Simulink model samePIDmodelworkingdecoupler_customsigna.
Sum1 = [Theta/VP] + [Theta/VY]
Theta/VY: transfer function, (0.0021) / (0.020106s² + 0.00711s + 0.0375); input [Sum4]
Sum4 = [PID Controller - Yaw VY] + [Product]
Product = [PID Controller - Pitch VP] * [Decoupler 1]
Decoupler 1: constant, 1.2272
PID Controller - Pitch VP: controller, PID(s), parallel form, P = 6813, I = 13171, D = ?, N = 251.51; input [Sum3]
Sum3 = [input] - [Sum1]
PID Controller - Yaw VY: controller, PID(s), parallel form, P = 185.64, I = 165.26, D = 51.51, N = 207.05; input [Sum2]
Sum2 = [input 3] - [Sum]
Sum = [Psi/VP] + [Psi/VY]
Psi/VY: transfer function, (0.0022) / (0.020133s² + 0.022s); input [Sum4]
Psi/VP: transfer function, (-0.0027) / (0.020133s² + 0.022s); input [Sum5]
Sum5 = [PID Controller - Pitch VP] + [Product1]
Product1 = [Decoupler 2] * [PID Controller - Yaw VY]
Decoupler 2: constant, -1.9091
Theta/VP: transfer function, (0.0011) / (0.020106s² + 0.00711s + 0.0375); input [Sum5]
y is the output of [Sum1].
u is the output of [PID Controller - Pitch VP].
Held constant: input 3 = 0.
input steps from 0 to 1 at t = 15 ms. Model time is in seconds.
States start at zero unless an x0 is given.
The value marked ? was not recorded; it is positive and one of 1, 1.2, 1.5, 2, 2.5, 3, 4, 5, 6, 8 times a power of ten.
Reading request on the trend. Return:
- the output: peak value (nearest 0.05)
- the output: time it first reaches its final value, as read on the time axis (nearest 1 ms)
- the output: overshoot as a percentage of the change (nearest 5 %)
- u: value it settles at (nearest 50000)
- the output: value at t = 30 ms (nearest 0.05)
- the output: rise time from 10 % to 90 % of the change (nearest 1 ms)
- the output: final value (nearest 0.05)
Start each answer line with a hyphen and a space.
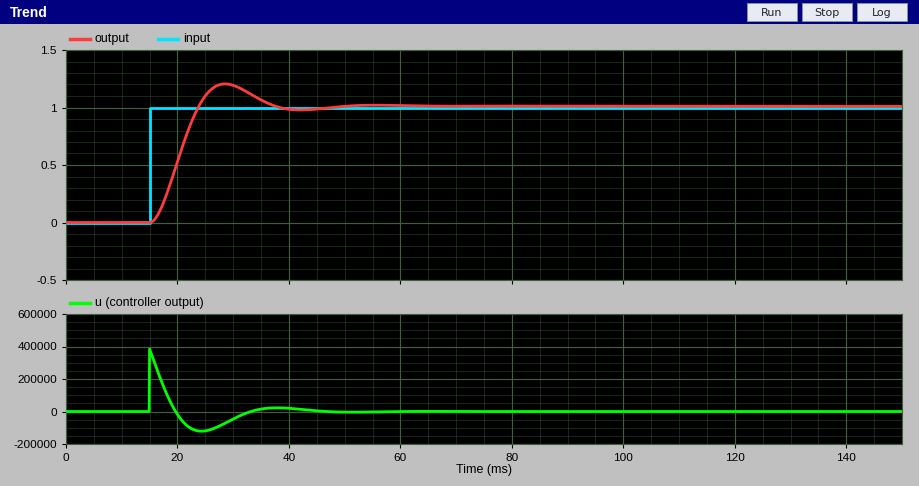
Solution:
- 1.20
- 24 ms
- 20 %
- 0
- 1.20
- 6 ms
- 1.00
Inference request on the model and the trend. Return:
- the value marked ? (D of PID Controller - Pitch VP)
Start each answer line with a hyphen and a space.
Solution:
- 1500
